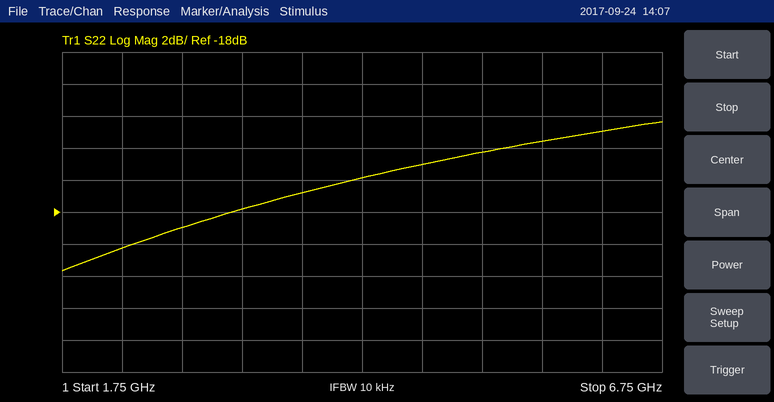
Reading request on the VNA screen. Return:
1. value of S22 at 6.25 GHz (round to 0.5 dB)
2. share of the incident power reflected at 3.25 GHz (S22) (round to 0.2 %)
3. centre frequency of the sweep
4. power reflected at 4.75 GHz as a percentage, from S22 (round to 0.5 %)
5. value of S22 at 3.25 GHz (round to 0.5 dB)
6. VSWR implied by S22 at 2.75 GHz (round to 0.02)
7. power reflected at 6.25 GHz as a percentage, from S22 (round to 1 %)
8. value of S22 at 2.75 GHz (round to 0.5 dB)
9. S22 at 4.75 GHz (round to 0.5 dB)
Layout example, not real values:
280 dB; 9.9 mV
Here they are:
-13.0 dB; 1.6 %; 4.25 GHz; 3.0 %; -18.0 dB; 1.26; 5 %; -19.0 dB; -15.0 dB
